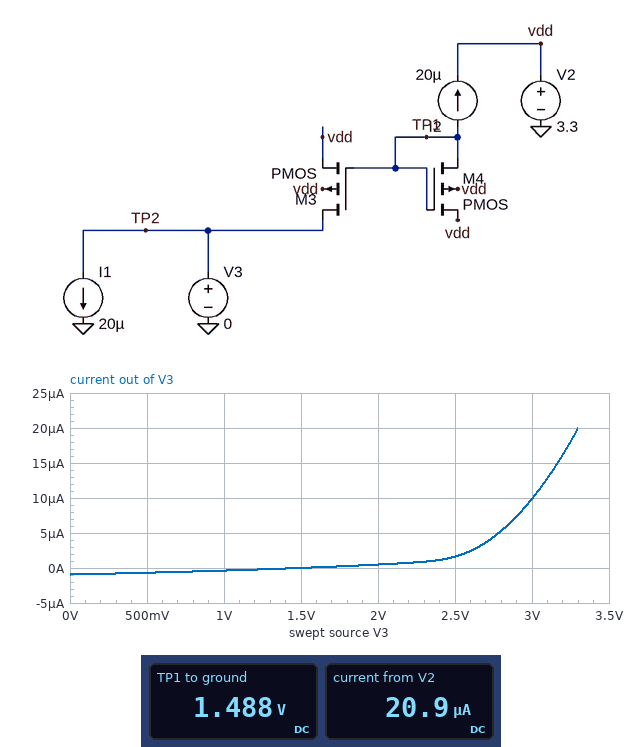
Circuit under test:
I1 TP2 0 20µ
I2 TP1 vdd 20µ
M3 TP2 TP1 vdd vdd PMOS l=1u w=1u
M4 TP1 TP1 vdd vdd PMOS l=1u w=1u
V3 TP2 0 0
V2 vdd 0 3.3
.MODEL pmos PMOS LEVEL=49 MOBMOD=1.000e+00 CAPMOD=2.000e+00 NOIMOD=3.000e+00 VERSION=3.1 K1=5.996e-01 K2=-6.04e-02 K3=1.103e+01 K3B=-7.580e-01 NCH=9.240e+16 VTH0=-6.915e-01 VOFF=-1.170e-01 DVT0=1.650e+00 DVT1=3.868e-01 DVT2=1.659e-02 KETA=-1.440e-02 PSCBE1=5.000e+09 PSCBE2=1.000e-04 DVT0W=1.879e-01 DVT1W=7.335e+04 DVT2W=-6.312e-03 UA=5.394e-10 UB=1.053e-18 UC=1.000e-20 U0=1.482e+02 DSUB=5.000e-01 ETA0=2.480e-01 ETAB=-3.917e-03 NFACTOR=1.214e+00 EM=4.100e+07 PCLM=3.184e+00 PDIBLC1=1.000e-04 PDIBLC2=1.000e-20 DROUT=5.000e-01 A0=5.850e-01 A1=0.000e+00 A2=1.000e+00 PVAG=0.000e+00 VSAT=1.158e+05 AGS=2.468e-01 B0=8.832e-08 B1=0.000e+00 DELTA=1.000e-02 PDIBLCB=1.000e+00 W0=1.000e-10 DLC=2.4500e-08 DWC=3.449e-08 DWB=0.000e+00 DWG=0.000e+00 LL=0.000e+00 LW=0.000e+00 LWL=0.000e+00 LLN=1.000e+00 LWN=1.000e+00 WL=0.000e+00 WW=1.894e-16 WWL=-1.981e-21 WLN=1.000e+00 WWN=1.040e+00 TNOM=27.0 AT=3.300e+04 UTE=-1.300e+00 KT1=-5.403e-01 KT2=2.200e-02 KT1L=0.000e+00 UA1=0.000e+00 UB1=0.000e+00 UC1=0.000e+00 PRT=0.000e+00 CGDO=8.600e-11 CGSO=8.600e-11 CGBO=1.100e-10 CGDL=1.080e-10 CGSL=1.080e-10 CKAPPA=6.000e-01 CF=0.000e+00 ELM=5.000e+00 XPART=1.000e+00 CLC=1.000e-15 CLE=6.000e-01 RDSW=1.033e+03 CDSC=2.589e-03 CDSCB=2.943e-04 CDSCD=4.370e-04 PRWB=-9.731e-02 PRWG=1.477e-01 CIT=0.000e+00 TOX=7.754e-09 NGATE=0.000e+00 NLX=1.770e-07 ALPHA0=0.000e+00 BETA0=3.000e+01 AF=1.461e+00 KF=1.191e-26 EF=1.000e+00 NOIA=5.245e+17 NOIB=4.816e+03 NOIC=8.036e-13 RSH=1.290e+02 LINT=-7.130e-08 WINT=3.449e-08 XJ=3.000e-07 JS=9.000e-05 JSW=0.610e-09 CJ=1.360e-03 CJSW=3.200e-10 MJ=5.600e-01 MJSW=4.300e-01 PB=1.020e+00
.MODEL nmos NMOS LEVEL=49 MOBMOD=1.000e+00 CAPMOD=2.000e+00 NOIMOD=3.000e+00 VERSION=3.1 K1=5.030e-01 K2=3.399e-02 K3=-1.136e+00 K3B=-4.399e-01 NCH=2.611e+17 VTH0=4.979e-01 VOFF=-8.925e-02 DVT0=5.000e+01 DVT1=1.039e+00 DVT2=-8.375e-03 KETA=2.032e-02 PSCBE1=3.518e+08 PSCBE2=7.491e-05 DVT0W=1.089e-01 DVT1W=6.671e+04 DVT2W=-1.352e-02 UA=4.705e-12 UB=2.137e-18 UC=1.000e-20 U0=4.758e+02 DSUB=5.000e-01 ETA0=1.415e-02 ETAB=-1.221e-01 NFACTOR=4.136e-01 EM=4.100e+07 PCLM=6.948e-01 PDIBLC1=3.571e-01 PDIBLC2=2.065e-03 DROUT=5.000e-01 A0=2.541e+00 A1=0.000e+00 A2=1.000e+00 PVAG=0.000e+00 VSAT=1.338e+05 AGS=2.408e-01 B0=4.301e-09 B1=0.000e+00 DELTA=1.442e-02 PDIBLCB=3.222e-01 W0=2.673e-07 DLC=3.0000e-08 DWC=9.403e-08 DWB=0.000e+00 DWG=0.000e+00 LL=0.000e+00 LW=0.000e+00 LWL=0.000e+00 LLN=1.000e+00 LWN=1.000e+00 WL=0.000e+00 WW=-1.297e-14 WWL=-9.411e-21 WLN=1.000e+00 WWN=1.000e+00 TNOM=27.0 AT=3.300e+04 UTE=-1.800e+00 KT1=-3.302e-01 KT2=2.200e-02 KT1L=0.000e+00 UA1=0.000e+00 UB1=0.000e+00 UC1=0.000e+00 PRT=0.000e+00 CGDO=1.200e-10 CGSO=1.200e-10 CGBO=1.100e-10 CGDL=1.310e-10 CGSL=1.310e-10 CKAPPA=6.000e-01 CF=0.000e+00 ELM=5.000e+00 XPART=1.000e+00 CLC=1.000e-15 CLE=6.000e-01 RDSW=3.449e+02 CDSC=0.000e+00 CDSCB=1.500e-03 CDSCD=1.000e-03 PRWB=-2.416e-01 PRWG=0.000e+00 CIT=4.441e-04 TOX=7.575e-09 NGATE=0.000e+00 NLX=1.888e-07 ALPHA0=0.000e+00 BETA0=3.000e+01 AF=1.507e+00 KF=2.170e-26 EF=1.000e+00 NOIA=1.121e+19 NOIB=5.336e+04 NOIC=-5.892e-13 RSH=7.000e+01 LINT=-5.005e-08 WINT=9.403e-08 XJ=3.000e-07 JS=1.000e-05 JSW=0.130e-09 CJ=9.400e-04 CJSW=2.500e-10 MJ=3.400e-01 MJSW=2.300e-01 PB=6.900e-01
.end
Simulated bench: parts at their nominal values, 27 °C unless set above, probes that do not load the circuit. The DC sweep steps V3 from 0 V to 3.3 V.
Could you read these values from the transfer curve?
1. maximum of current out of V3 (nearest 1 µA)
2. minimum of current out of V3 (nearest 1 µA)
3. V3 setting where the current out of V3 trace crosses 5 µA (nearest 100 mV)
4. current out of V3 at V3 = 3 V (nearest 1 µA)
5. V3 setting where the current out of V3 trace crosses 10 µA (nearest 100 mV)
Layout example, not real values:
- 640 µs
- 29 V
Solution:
- 20 µA
- -1 µA
- 2.8 V
- 10 µA
- 3.0 V
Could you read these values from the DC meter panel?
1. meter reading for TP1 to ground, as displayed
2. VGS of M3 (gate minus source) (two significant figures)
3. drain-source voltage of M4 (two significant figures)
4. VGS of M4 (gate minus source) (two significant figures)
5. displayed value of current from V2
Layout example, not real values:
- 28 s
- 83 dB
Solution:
- 1.488 V
- -1.8 V
- -1.8 V
- -1.8 V
- 20.9 µA
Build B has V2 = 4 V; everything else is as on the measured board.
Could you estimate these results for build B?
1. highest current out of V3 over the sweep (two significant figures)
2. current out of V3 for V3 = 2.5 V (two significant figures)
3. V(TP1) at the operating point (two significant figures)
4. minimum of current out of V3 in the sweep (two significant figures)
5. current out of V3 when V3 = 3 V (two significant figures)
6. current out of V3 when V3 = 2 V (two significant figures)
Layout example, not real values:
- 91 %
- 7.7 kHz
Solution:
- 2.4 µA
- 280 nA
- 2.2 V
- -1.2 µA
- 900 nA
- -150 nA
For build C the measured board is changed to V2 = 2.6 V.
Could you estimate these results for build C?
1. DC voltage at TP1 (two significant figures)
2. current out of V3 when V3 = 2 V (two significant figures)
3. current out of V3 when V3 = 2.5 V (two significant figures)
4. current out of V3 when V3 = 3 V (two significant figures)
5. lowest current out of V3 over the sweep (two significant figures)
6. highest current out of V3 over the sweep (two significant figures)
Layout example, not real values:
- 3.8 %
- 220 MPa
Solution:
- 790 mV
- 3.7 µA
- 16 µA
- 39 µA
- -560 nA
- 77 µA
